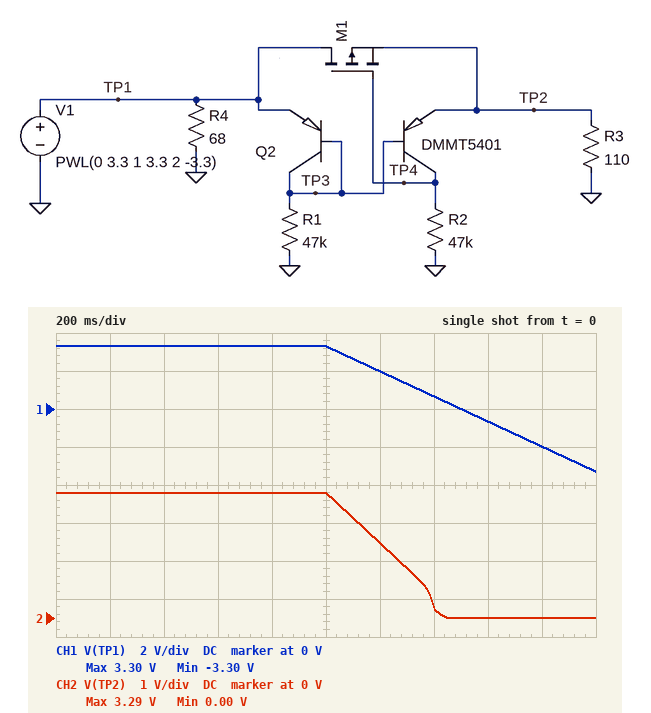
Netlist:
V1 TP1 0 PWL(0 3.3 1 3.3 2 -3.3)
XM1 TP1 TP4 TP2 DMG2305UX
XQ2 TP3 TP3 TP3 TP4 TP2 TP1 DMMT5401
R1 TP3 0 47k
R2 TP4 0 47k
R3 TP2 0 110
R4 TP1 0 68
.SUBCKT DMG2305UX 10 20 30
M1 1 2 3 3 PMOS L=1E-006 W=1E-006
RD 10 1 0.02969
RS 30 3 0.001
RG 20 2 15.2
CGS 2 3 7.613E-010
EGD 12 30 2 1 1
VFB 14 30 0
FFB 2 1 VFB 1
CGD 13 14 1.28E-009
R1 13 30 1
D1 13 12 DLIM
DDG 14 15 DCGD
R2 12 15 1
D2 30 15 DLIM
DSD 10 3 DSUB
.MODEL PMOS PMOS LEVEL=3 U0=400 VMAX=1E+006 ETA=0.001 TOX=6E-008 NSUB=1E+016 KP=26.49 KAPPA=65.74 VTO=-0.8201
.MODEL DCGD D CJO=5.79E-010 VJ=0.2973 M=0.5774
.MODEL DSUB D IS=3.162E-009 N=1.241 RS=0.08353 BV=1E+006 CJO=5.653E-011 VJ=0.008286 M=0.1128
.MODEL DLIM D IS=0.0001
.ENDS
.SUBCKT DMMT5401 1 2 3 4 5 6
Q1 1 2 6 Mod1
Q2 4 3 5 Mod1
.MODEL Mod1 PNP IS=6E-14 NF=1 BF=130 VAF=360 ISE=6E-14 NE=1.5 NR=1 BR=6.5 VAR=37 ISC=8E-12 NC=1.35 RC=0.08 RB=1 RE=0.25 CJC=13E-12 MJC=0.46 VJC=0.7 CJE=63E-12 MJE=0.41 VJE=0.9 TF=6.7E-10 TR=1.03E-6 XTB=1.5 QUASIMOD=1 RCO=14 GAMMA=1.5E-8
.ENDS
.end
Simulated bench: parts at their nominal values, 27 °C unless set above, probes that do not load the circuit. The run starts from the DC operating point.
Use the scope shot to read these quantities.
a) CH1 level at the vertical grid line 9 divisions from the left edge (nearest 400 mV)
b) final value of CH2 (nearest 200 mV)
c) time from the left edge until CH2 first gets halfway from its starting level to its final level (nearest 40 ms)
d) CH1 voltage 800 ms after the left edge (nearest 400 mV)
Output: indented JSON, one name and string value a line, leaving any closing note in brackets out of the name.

{
  "CH1 level at the vertical grid line 9 divisions from the left edge": "-2.0 V",
  "final value of CH2": "0 V",
  "time from the left edge until CH2 first gets halfway from its starting level to its final level": "1.24 s",
  "CH1 voltage 800 ms after the left edge": "3.2 V"
}
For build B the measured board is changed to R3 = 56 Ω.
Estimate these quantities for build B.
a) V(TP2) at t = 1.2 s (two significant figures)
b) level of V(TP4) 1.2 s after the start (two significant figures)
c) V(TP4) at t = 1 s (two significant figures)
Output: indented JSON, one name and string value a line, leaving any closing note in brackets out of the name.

{
  "V(TP2) at t = 1.2 s": "2.0 V",
  "level of V(TP4) 1.2 s after the start": "1.0 V",
  "V(TP4) at t = 1 s": "2.1 V"
}
